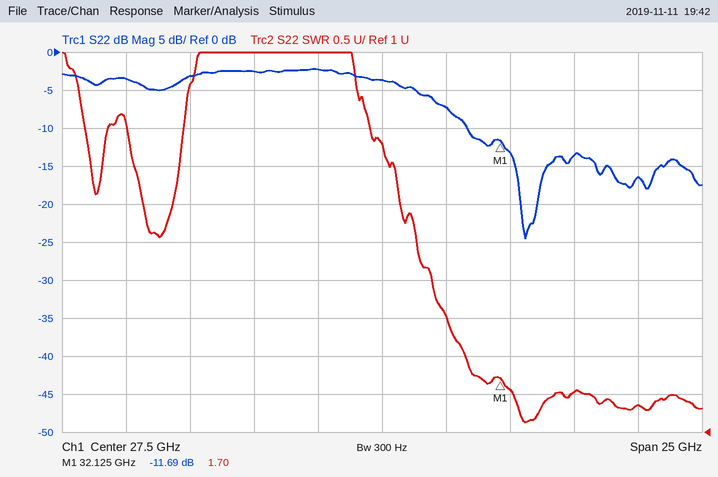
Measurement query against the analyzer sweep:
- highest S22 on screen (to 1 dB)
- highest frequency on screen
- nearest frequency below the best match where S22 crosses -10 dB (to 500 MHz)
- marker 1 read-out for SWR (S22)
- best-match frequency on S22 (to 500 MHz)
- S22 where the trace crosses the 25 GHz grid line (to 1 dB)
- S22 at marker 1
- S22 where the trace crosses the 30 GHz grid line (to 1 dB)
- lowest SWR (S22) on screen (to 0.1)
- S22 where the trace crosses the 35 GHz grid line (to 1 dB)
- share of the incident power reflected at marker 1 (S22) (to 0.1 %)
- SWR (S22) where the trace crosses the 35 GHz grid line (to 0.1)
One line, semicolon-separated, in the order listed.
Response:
-2 dB; 40 GHz; 31.0 GHz; 1.70; 33.0 GHz; -2 dB; -11.69 dB; -7 dB; 1.1; -14 dB; 6.8 %; 1.5
